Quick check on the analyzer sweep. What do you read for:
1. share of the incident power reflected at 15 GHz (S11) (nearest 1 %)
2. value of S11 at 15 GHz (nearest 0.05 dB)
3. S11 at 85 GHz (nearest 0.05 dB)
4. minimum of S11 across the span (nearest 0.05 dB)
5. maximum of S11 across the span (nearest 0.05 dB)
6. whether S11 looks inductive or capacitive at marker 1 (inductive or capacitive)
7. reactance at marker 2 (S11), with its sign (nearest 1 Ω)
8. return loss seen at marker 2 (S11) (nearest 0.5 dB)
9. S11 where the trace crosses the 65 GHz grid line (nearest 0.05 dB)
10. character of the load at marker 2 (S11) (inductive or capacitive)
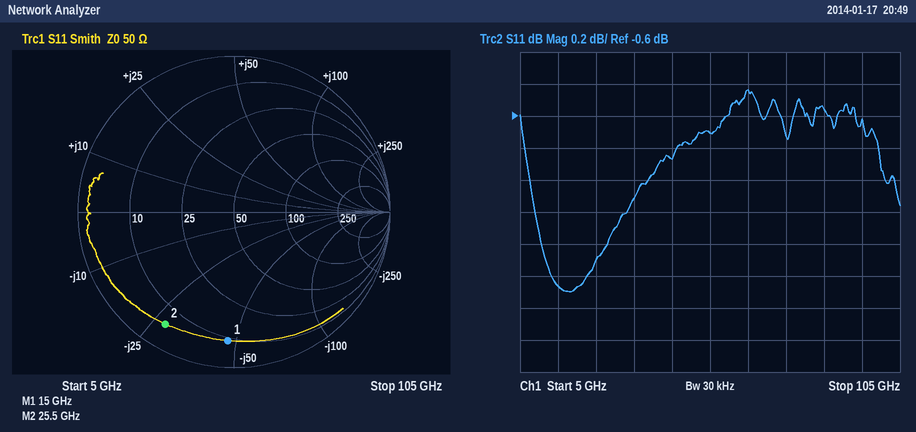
68 %
-1.65 dB
-0.55 dB
-1.70 dB
-0.45 dB
capacitive
-28 Ω
1.5 dB
-0.45 dB
capacitive
